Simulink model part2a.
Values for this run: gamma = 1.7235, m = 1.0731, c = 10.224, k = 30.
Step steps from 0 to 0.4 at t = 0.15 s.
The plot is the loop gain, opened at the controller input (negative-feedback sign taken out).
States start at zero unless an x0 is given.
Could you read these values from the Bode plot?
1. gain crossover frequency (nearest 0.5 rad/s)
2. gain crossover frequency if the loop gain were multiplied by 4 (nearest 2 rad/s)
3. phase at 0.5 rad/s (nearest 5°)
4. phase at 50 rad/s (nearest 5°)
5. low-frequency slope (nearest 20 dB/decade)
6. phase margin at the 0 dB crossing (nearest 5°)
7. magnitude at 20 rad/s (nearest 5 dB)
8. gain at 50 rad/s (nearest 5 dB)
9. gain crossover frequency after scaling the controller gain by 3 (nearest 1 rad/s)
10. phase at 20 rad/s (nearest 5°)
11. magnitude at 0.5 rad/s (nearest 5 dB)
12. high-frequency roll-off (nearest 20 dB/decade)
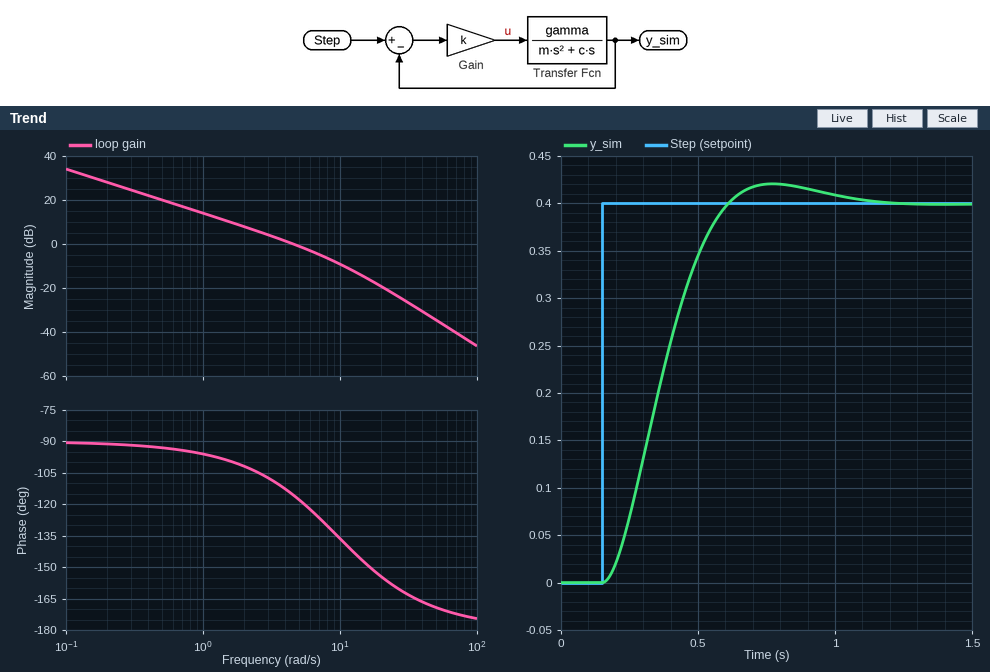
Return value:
4.5 rad/s
12 rad/s
-95°
-170°
-20 dB/decade
65°
-20 dB
-35 dB
10 rad/s
-155°
20 dB
-40 dB/decade
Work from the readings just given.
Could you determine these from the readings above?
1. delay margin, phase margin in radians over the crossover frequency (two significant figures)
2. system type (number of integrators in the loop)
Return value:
0.25 s
1
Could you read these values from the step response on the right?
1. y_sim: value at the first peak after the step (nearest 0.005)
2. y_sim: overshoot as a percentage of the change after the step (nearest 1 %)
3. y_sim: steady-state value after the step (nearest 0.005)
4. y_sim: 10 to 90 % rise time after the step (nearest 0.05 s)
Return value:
0.420
5 %
0.400
0.30 s
